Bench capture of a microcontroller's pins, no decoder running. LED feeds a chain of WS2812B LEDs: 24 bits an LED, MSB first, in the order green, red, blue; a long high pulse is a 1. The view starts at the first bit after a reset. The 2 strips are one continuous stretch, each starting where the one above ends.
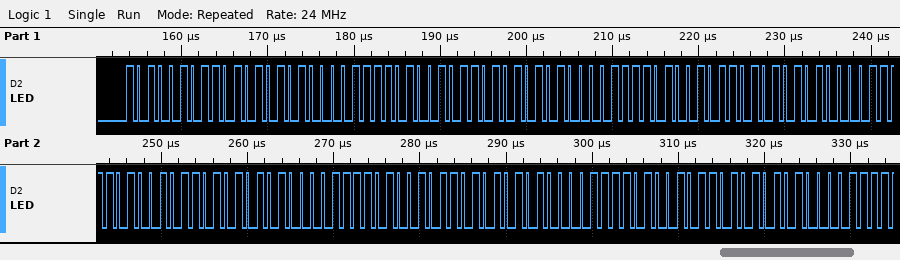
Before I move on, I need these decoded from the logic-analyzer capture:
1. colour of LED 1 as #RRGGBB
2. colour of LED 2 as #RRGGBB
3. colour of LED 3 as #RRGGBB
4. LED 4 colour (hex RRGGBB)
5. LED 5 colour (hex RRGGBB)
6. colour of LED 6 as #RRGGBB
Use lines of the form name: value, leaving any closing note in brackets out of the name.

colour of LED 1 as #RRGGBB: #AAA587
colour of LED 2 as #RRGGBB: #AAA587
colour of LED 3 as #RRGGBB: #AAA587
LED 4 colour: #AAA587
LED 5 colour: #AAA587
colour of LED 6 as #RRGGBB: #AAA587
